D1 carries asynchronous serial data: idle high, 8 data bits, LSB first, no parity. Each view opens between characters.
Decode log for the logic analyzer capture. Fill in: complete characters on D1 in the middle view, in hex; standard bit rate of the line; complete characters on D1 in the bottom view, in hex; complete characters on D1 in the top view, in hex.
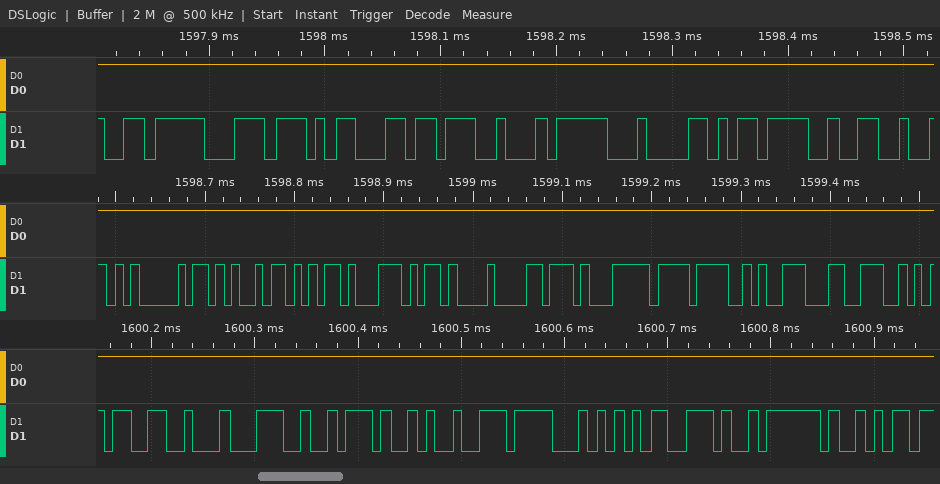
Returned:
05, 2B, AB, 71, 0B, D8, F1, EF, CA, CC
115200 baud
33, C4, D2, 29, EE, 54, 73, FA, A9
F6, DC, 8D, 3B, F4, 84, ED, 32
